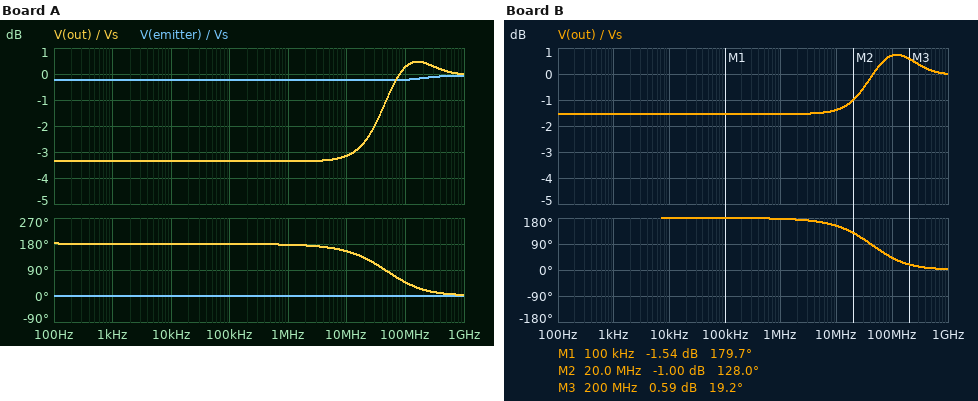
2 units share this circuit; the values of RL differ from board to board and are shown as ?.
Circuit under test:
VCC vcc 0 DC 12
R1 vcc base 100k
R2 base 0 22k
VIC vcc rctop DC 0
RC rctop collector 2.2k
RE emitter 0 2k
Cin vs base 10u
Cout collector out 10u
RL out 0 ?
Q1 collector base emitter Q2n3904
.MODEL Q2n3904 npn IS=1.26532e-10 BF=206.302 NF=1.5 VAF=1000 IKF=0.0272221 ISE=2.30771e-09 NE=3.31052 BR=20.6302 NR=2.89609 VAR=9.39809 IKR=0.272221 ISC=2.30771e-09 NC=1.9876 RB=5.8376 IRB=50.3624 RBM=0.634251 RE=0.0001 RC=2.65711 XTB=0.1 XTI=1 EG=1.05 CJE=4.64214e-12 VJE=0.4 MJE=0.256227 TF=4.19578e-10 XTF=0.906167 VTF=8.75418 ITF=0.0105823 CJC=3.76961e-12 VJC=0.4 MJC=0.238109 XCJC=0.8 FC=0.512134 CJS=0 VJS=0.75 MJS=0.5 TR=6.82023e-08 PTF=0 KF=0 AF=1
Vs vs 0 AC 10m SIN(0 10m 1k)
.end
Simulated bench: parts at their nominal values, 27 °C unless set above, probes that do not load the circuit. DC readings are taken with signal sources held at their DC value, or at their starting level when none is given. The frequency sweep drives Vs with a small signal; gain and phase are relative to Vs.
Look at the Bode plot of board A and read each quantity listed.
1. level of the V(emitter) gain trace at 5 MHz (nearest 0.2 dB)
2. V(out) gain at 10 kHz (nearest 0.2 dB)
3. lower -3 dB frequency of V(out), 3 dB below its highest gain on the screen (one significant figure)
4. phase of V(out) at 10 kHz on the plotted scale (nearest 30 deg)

-0.2 dB
-3.4 dB
20 MHz
180 deg
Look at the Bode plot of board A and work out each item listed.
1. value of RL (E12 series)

3.9 kΩ
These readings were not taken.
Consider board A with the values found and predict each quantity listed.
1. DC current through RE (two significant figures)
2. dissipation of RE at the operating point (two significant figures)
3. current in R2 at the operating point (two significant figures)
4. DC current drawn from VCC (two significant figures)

720 µA
1.0 mW
93 µA
810 µA
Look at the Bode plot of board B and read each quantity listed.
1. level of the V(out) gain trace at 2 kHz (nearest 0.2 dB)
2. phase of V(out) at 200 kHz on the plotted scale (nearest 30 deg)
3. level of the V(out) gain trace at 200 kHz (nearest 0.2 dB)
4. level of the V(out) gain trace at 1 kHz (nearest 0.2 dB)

-1.6 dB
180 deg
-1.6 dB
-1.6 dB
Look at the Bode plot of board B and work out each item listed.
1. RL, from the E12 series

8.2 kΩ
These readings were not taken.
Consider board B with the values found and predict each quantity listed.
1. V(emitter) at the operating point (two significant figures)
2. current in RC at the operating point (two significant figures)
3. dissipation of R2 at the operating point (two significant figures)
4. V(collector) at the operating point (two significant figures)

1.4 V
710 µA
190 µW
10 V
